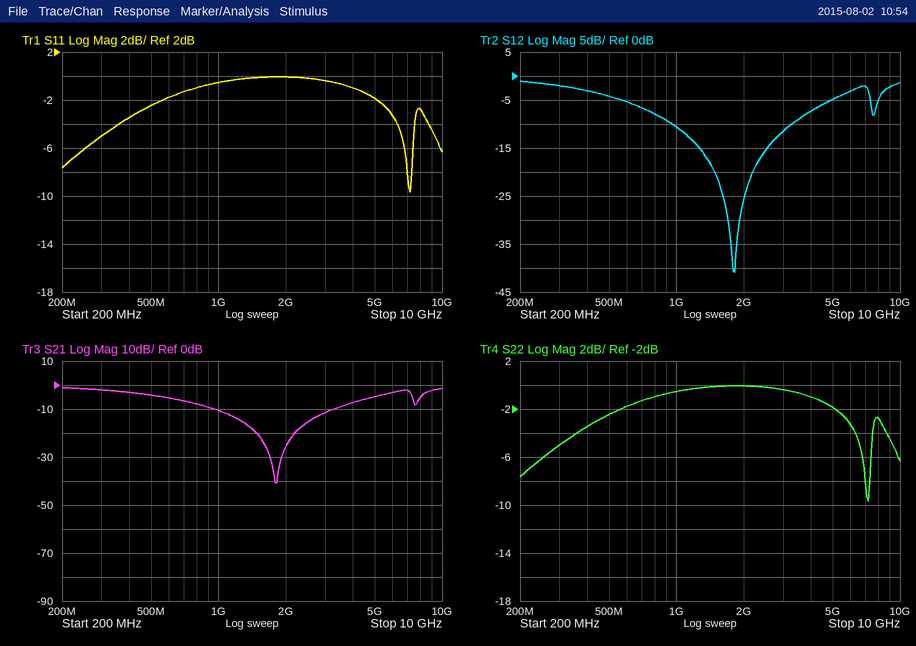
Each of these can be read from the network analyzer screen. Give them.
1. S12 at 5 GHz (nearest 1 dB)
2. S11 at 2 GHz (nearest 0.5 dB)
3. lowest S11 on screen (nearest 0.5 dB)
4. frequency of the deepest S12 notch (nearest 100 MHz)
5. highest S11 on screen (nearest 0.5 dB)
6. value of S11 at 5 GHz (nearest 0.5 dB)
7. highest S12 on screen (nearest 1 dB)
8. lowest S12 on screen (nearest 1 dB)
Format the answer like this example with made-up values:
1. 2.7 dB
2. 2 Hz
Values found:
1. -5 dB
2. 0.0 dB
3. -9.5 dB
4. 1.8 GHz
5. 0.0 dB
6. -2.0 dB
7. -1 dB
8. -41 dB
